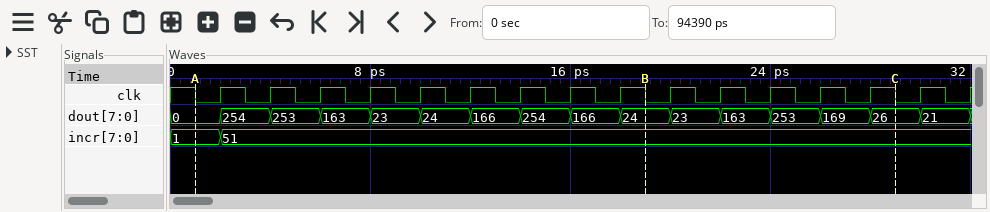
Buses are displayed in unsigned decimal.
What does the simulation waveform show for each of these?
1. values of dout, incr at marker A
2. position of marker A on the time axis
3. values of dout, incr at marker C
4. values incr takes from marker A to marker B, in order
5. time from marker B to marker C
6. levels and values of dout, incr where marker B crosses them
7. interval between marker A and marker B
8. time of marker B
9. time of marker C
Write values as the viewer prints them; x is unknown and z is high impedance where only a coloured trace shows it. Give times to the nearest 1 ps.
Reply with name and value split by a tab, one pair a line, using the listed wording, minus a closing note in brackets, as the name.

values of dout, incr at marker A	dout=0, incr=1
position of marker A on the time axis	1 ps
values of dout, incr at marker C	dout=26, incr=51
values incr takes from marker A to marker B, in order	1, 51
time from marker B to marker C	10 ps
levels and values of dout, incr where marker B crosses them	dout=24, incr=51
interval between marker A and marker B	18 ps
time of marker B	19 ps
time of marker C	29 ps
